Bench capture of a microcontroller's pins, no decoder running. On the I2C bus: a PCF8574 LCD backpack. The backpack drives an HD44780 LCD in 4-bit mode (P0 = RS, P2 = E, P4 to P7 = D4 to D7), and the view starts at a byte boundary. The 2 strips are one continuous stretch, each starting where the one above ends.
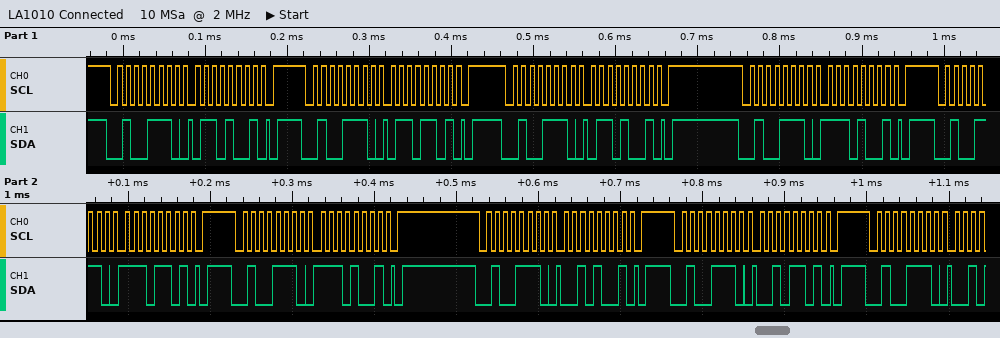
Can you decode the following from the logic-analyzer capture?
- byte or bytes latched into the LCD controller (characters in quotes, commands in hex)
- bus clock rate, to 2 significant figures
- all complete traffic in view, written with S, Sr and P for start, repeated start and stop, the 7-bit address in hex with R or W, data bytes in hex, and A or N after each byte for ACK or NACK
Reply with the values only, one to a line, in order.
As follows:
'n'
100 kHz
S 27W A 69 A P S 27W A 6D A P S 27W A 69 A P S 27W A E9 A P S 27W A ED A P S 27W A E9 A P S 27W A 29 A P S 27W A 2D A P S 27W A
